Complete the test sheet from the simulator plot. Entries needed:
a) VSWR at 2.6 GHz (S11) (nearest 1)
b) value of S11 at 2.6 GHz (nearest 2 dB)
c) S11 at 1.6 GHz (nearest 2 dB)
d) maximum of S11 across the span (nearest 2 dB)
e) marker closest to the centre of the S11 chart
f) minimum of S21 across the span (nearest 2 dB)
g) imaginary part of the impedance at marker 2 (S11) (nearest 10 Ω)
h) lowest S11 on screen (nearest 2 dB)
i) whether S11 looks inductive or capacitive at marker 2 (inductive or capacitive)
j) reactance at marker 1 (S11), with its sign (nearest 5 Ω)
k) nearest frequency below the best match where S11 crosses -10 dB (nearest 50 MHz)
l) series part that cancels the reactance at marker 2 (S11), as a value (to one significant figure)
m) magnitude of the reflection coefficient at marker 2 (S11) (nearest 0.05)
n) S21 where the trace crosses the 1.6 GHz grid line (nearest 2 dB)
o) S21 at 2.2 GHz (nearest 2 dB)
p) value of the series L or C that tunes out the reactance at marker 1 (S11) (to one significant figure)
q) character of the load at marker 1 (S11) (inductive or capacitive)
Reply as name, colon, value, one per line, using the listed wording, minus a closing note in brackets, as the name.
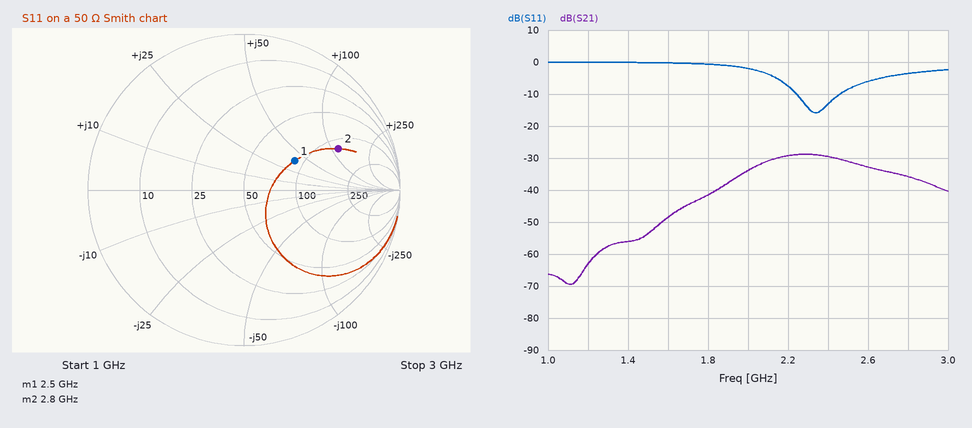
VSWR at 2.6 GHz (S11): 3
value of S11 at 2.6 GHz: -6 dB
S11 at 1.6 GHz: 0 dB
maximum of S11 across the span: 0 dB
marker closest to the centre of the S11 chart: marker 1
minimum of S21 across the span: -70 dB
imaginary part of the impedance at marker 2 (S11): +120 Ω
lowest S11 on screen: -16 dB
whether S11 looks inductive or capacitive at marker 2: inductive
reactance at marker 1 (S11), with its sign: +40 Ω
nearest frequency below the best match where S11 crosses -10 dB: 2.25 GHz
series part that cancels the reactance at marker 2 (S11), as a value: 500 fF
magnitude of the reflection coefficient at marker 2 (S11): 0.65
S21 where the trace crosses the 1.6 GHz grid line: -48 dB
S21 at 2.2 GHz: -30 dB
value of the series L or C that tunes out the reactance at marker 1 (S11): 2 pF
character of the load at marker 1 (S11): inductive
